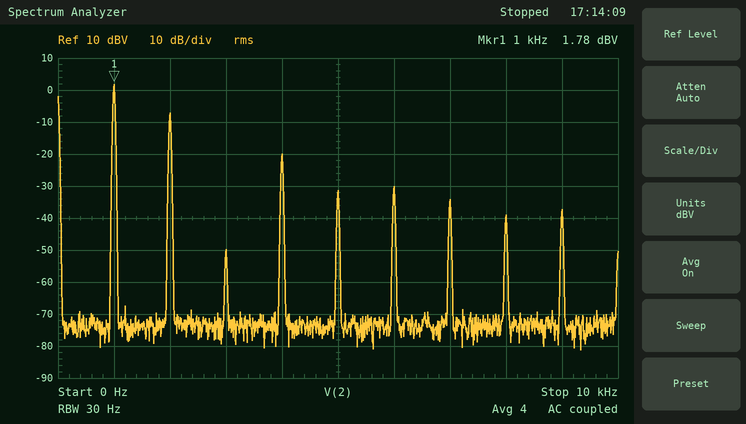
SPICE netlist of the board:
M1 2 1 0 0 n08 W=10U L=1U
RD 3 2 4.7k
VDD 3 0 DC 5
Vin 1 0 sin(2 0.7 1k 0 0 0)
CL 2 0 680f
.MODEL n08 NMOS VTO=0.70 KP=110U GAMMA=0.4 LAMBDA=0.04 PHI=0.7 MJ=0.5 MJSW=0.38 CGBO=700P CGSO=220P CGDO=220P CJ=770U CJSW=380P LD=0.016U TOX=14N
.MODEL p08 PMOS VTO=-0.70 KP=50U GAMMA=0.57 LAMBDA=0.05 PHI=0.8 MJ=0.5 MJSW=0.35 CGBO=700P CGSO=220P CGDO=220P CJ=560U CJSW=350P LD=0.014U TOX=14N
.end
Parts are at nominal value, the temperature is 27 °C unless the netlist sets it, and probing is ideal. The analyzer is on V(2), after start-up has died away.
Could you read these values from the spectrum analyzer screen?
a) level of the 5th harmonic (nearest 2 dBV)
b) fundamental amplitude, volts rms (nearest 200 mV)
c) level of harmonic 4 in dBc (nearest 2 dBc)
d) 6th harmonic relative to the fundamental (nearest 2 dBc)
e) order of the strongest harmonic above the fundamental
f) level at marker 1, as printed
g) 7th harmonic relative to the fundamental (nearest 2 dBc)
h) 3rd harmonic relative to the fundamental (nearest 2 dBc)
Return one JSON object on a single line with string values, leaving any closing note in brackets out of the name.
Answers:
{"level of the 5th harmonic": "-32 dBV", "fundamental amplitude, volts rms": "1.2 V", "level of harmonic 4 in dBc": "-22 dBc", "6th harmonic relative to the fundamental": "-32 dBc", "order of the strongest harmonic above the fundamental": "2", "level at marker 1, as printed": "1.78 dBV", "7th harmonic relative to the fundamental": "-36 dBc", "3rd harmonic relative to the fundamental": "-52 dBc"}
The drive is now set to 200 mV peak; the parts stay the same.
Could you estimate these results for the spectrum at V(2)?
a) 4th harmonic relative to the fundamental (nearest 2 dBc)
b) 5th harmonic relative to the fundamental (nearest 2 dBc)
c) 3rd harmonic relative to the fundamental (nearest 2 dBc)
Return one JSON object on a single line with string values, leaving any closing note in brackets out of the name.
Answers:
{"4th harmonic relative to the fundamental": "-34 dBc", "5th harmonic relative to the fundamental": "-36 dBc", "3rd harmonic relative to the fundamental": "-18 dBc"}
